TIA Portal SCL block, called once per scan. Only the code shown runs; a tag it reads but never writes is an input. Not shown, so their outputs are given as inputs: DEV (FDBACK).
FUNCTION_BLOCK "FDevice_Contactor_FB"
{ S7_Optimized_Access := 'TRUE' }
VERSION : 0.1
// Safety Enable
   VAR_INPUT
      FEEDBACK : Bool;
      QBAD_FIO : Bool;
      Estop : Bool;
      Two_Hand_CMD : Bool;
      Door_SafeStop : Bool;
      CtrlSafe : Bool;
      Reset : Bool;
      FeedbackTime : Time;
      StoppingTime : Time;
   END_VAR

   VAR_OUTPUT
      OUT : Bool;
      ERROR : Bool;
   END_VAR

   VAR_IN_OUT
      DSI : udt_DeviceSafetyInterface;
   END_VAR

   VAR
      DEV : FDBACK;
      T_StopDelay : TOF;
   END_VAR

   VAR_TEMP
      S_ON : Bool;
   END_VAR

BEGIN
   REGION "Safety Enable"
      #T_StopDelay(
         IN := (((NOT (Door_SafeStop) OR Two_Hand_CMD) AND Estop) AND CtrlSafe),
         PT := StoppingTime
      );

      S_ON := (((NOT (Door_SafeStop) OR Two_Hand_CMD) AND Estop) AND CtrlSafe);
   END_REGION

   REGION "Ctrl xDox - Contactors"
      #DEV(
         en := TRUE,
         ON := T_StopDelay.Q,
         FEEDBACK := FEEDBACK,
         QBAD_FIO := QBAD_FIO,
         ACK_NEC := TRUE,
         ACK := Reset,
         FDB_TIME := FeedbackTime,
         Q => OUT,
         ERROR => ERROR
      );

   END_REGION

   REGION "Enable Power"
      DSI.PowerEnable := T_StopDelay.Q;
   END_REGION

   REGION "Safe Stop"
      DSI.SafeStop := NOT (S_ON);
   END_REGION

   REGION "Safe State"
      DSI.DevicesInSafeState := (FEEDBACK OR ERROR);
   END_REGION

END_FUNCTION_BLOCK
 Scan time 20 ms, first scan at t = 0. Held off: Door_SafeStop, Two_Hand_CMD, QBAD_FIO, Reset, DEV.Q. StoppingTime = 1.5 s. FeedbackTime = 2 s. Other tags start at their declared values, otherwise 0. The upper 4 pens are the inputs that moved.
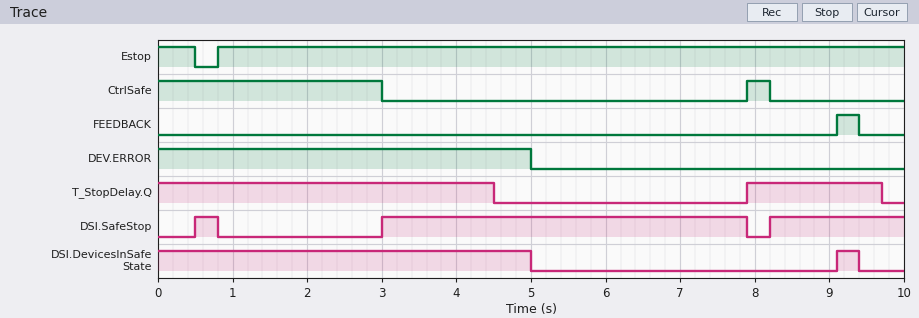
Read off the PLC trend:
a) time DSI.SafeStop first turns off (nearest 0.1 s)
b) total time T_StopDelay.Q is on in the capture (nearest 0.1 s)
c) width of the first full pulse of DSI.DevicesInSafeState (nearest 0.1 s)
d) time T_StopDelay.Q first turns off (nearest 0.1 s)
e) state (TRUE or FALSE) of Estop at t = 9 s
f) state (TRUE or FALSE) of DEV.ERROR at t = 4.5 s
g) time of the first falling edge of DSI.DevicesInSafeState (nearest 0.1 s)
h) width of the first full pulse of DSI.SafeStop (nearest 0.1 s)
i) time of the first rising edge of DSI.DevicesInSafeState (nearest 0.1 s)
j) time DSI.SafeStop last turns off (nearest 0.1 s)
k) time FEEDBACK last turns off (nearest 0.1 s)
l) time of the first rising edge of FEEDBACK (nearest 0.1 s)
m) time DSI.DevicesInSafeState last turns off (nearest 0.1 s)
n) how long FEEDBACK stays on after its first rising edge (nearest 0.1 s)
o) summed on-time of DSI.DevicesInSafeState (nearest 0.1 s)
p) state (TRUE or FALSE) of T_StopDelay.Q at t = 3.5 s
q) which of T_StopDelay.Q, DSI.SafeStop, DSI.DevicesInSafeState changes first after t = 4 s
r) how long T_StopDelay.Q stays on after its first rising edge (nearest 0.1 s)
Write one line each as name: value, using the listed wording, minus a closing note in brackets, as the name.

time DSI.SafeStop first turns off: 0.8 s
total time T_StopDelay.Q is on in the capture: 6.3 s
width of the first full pulse of DSI.DevicesInSafeState: 0.3 s
time T_StopDelay.Q first turns off: 4.5 s
state (TRUE or FALSE) of Estop at t = 9 s: TRUE
state (TRUE or FALSE) of DEV.ERROR at t = 4.5 s: TRUE
time of the first falling edge of DSI.DevicesInSafeState: 5.0 s
width of the first full pulse of DSI.SafeStop: 0.3 s
time of the first rising edge of DSI.DevicesInSafeState: 9.1 s
time DSI.SafeStop last turns off: 7.9 s
time FEEDBACK last turns off: 9.4 s
time of the first rising edge of FEEDBACK: 9.1 s
time DSI.DevicesInSafeState last turns off: 9.4 s
how long FEEDBACK stays on after its first rising edge: 0.3 s
summed on-time of DSI.DevicesInSafeState: 5.3 s
state (TRUE or FALSE) of T_StopDelay.Q at t = 3.5 s: TRUE
which of T_StopDelay.Q, DSI.SafeStop, DSI.DevicesInSafeState changes first after t = 4 s: T_StopDelay.Q
how long T_StopDelay.Q stays on after its first rising edge: 1.8 s
